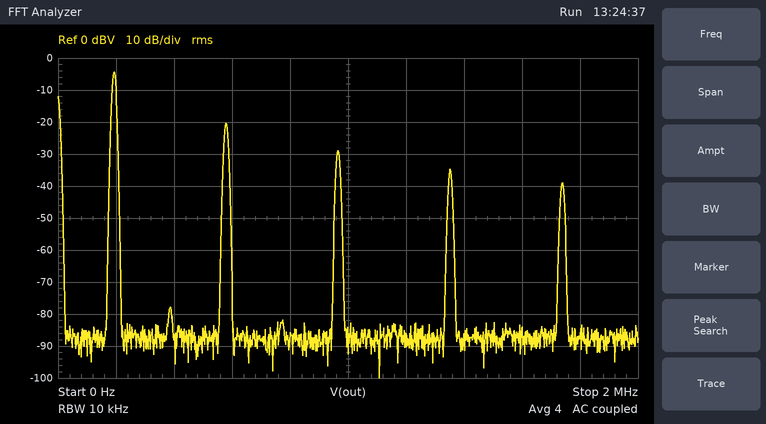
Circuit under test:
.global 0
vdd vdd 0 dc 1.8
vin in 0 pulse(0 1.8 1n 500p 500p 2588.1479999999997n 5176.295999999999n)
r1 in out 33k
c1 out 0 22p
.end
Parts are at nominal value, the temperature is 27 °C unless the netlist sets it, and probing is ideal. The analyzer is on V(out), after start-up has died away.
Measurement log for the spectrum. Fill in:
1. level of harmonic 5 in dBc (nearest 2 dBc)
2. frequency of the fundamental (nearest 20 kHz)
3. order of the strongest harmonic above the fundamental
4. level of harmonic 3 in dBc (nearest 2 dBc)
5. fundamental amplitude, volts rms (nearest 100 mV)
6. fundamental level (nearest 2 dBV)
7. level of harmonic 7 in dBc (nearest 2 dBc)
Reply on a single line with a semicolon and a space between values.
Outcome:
-24 dBc; 200 kHz; 3; -16 dBc; 600 mV; -4 dBV; -30 dBc
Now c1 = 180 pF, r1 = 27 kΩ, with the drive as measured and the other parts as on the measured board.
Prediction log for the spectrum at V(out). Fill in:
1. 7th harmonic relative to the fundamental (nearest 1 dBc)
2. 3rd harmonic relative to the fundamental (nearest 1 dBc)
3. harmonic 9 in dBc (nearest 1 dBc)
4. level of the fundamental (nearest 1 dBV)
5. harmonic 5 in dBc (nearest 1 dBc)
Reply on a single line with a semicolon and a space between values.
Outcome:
-34 dBc; -19 dBc; -38 dBc; -17 dBV; -28 dBc
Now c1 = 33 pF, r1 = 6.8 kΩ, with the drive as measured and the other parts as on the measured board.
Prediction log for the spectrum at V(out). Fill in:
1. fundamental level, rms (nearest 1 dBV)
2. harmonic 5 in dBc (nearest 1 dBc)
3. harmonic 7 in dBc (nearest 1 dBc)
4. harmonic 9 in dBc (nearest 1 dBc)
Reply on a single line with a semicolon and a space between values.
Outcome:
-2 dBV; -18 dBc; -23 dBc; -27 dBc
